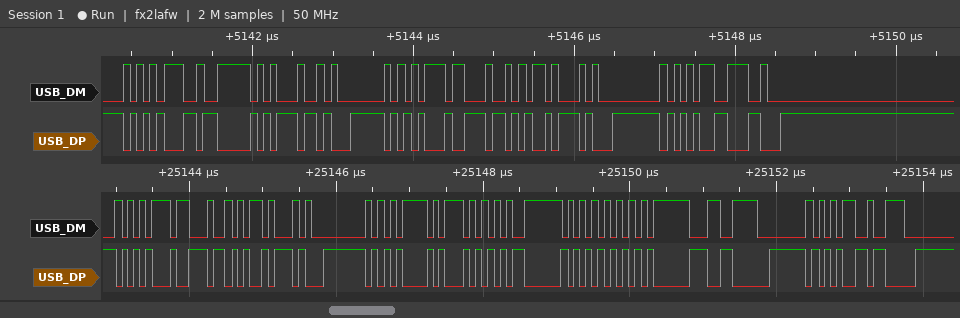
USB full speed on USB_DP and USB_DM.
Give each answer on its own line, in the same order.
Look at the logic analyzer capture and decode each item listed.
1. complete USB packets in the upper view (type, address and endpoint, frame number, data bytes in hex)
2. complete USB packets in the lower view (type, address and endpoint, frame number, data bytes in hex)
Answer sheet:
SOF 775, IN ADDR 2 EP 1, NAK
IN ADDR 2 EP 1, DATA0 [ 00 FA 00 00 ], ACK
